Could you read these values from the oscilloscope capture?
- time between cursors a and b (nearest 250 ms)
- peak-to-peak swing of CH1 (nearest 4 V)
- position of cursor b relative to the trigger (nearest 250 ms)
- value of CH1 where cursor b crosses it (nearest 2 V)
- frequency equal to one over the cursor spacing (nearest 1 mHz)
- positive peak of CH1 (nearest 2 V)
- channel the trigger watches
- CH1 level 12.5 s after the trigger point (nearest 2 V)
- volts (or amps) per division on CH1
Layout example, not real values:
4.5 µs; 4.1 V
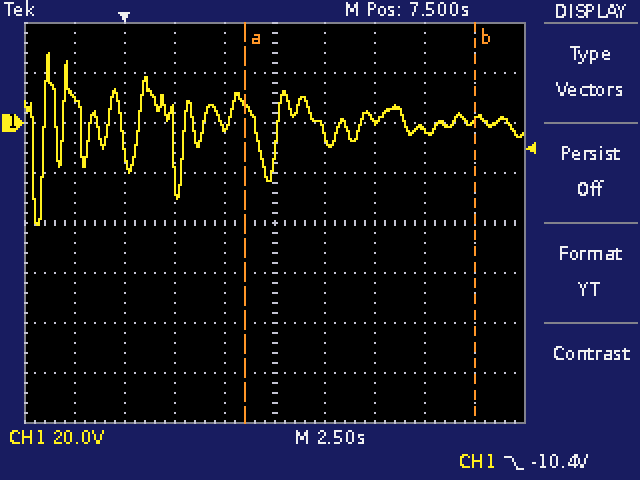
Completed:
11.50 s; 68 V; +17.50 s; 2 V; 87 mHz; 28 V; CH1; 2 V; 20 V
